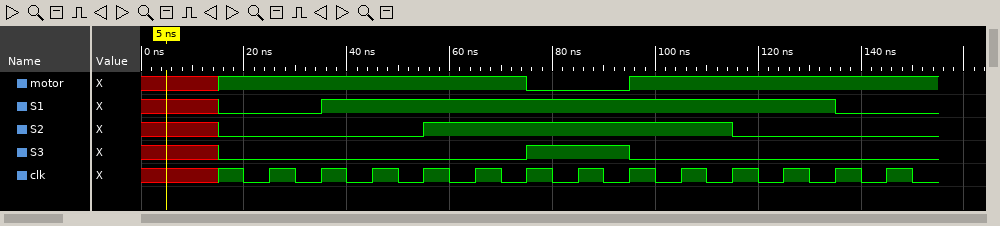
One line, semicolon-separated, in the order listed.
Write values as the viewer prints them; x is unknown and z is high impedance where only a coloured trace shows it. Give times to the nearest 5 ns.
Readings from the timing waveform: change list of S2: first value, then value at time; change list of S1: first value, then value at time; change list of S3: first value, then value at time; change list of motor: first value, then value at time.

x, 0 at 15 ns, 1 at 55 ns, 0 at 115 ns; x, 0 at 15 ns, 1 at 35 ns, 0 at 135 ns; x, 0 at 15 ns, 1 at 75 ns, 0 at 95 ns; x, 1 at 15 ns, 0 at 75 ns, 1 at 95 ns
